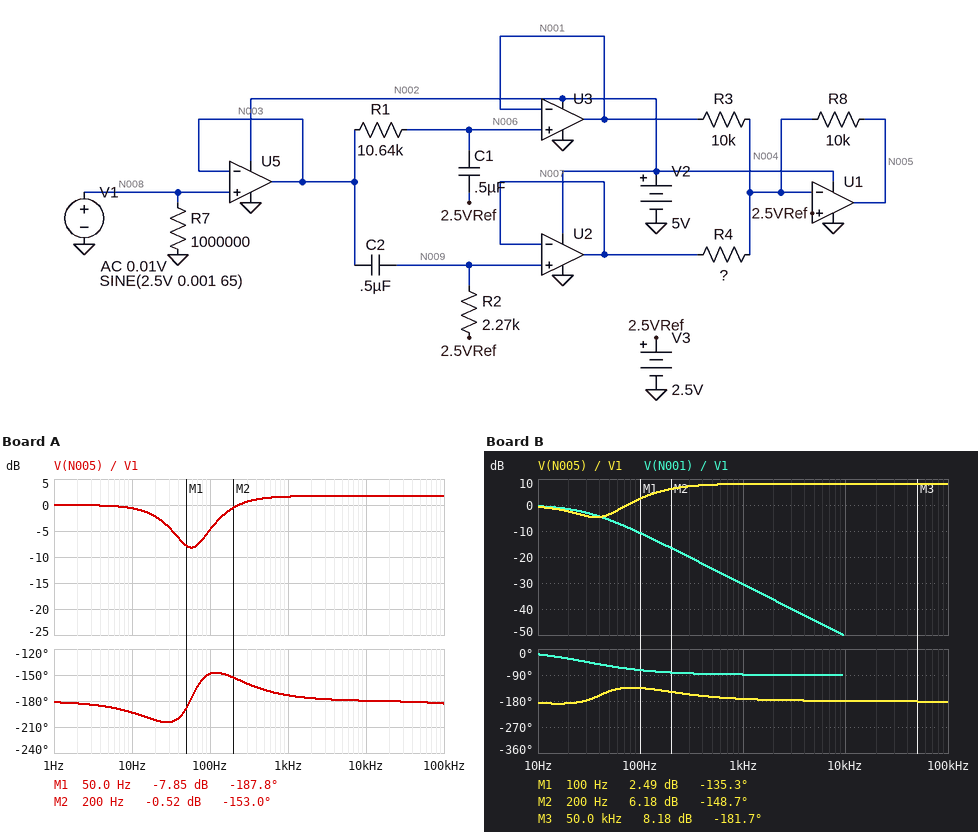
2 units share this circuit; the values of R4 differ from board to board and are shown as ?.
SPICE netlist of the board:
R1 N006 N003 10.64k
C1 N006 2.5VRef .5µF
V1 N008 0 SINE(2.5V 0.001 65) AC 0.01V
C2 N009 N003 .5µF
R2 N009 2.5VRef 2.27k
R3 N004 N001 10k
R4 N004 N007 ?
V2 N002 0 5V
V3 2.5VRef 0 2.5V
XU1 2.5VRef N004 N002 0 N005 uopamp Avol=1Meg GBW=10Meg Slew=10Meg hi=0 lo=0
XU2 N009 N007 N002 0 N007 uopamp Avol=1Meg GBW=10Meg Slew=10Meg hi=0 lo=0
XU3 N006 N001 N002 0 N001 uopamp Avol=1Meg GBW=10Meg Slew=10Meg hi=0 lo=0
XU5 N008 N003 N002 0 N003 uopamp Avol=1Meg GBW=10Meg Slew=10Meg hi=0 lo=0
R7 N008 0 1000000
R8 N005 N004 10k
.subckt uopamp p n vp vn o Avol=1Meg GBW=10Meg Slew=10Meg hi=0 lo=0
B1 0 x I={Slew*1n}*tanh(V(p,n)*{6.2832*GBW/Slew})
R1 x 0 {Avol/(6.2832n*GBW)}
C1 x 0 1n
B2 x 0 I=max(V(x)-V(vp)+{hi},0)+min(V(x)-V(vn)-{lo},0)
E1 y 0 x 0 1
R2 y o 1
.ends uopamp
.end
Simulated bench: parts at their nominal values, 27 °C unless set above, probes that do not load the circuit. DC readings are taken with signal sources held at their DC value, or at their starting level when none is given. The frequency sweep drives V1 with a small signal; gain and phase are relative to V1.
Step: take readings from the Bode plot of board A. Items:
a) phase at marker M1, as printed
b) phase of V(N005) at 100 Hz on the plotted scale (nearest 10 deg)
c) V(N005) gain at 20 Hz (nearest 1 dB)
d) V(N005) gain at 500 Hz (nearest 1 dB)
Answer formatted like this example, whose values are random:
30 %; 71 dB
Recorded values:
-187.8 deg; -150 deg; -2 dB; 1 dB
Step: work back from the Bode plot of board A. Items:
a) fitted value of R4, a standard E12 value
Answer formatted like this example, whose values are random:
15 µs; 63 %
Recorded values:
8.2 kΩ
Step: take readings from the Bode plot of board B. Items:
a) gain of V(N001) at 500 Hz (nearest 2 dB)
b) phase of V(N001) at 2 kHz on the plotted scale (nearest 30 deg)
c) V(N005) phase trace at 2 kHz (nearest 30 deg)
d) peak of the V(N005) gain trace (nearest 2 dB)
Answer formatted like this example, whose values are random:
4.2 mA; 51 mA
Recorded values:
-24 dB; -90 deg; -180 deg; 8 dB
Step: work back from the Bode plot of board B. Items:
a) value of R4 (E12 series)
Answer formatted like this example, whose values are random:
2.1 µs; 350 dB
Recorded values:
3.9 kΩ
